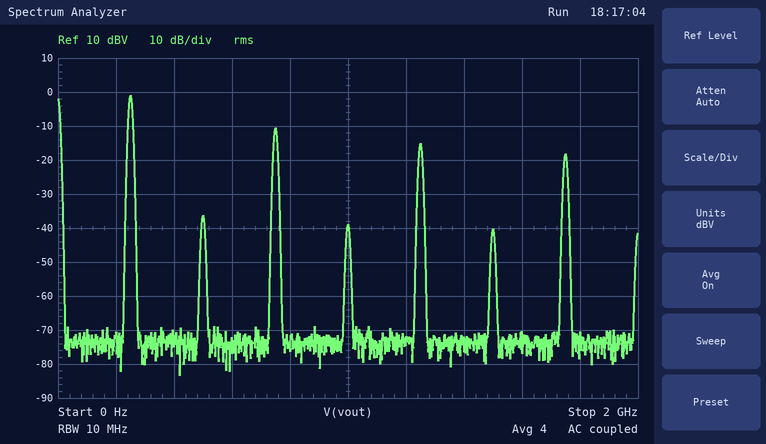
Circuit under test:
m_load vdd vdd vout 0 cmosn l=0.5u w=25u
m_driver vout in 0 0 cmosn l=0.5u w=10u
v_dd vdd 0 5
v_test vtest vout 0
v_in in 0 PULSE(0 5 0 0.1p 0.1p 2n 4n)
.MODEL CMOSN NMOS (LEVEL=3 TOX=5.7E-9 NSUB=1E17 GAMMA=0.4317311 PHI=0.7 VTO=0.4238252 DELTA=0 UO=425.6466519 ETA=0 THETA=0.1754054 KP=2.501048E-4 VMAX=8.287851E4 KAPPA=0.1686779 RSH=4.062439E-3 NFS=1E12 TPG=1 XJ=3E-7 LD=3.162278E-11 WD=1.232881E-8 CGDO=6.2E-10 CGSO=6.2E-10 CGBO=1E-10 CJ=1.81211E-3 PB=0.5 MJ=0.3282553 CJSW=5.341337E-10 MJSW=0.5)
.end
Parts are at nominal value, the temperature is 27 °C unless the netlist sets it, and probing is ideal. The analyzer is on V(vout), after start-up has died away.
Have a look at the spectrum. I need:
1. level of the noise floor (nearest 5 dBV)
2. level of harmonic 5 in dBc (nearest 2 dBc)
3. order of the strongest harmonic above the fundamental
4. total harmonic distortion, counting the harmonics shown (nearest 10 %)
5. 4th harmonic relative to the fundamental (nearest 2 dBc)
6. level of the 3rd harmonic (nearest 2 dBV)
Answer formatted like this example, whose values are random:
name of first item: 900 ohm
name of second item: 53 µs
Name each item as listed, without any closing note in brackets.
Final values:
level of the noise floor: -75 dBV
level of harmonic 5 in dBc: -14 dBc
order of the strongest harmonic above the fundamental: 3
total harmonic distortion, counting the harmonics shown: 40 %
4th harmonic relative to the fundamental: -38 dBc
level of the 3rd harmonic: -10 dBV
